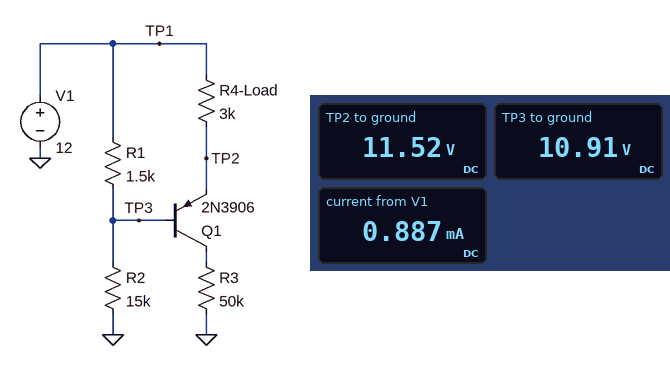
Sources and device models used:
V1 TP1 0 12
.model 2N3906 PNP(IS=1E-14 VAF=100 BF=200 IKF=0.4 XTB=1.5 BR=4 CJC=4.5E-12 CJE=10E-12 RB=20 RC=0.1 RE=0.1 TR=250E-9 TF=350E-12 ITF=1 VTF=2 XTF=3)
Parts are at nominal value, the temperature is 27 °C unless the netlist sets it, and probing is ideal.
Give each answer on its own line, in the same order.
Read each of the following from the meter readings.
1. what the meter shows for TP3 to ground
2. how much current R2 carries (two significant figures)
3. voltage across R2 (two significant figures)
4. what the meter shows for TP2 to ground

10.91 V
730 µA
11 V
11.52 V
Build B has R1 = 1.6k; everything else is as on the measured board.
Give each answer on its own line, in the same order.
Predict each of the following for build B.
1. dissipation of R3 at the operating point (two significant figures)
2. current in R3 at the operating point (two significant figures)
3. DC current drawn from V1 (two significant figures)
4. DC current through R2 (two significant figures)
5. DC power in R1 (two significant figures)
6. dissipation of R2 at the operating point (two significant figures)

1.6 mW
180 µA
900 µA
720 µA
830 µW
7.8 mW
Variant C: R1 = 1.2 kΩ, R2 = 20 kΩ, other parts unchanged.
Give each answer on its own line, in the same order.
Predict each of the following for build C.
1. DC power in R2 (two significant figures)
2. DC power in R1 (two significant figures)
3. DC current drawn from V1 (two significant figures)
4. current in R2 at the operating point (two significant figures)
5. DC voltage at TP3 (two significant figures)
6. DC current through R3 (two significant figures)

6.4 mW
380 µW
600 µA
570 µA
11 V
37 µA
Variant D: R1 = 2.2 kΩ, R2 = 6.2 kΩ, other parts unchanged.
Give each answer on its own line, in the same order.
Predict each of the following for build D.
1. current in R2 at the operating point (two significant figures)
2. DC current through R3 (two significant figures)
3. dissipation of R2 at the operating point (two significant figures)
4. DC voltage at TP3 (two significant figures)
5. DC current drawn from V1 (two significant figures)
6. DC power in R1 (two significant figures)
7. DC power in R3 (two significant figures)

1.5 mA
200 µA
15 mW
9.5 V
1.7 mA
2.8 mW
2.1 mW
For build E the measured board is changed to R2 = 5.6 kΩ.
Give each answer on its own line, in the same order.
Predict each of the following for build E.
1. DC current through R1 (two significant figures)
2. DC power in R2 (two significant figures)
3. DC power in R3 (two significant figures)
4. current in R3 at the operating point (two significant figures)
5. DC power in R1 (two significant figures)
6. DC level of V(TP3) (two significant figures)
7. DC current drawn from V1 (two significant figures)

1.5 mA
17 mW
2.2 mW
210 µA
3.2 mW
9.8 V
2.0 mA
